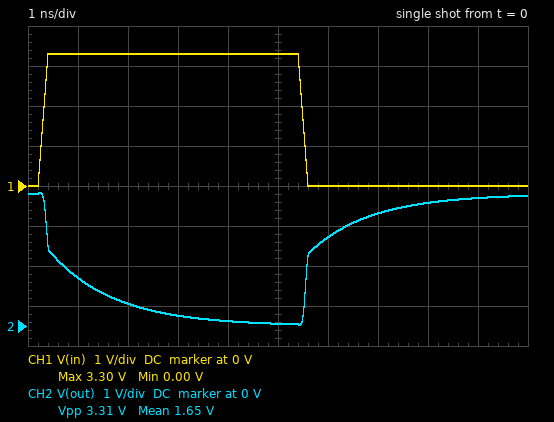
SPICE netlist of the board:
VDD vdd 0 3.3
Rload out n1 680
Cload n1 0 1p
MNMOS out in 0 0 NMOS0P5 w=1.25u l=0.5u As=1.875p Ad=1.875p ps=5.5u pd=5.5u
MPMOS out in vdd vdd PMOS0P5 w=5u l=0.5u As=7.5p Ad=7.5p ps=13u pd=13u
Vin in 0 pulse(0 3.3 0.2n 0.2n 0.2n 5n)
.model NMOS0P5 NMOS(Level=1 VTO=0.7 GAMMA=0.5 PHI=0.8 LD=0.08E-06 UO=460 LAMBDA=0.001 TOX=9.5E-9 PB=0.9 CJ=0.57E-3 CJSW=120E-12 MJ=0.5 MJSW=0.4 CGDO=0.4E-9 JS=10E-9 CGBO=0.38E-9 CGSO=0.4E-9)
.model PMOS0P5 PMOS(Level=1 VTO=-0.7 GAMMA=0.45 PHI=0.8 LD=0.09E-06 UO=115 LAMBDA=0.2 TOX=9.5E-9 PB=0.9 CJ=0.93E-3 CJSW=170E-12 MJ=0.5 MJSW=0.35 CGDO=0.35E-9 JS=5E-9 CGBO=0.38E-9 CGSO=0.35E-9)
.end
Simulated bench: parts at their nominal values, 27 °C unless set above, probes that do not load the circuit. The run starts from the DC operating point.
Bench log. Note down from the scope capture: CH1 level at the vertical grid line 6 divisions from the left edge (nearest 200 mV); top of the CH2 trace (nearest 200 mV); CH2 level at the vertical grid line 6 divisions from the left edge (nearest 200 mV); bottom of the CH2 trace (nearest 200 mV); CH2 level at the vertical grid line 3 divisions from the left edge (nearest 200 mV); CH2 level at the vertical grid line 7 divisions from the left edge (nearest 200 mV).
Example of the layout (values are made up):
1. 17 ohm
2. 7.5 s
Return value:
1. 0 V
2. 3.4 V
3. 2.2 V
4. 0 V
5. 200 mV
6. 2.8 V
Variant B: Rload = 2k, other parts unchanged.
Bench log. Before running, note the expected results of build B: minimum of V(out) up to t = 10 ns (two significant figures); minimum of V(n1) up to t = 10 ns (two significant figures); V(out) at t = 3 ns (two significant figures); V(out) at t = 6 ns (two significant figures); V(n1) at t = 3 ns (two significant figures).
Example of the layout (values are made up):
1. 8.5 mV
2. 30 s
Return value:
1. 100 mV
2. 490 mV
3. 310 mV
4. 2.8 V
5. 1.2 V
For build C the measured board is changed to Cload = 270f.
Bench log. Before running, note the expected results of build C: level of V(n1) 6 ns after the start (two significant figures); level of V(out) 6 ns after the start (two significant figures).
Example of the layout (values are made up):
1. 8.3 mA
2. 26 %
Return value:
1. 2.4 V
2. 2.9 V
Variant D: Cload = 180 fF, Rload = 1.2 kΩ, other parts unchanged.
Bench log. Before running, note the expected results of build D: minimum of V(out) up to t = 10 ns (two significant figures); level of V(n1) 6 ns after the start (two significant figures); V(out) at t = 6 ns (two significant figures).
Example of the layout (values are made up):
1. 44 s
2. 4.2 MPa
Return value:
1. -26 mV
2. 2.5 V
3. 3.0 V
